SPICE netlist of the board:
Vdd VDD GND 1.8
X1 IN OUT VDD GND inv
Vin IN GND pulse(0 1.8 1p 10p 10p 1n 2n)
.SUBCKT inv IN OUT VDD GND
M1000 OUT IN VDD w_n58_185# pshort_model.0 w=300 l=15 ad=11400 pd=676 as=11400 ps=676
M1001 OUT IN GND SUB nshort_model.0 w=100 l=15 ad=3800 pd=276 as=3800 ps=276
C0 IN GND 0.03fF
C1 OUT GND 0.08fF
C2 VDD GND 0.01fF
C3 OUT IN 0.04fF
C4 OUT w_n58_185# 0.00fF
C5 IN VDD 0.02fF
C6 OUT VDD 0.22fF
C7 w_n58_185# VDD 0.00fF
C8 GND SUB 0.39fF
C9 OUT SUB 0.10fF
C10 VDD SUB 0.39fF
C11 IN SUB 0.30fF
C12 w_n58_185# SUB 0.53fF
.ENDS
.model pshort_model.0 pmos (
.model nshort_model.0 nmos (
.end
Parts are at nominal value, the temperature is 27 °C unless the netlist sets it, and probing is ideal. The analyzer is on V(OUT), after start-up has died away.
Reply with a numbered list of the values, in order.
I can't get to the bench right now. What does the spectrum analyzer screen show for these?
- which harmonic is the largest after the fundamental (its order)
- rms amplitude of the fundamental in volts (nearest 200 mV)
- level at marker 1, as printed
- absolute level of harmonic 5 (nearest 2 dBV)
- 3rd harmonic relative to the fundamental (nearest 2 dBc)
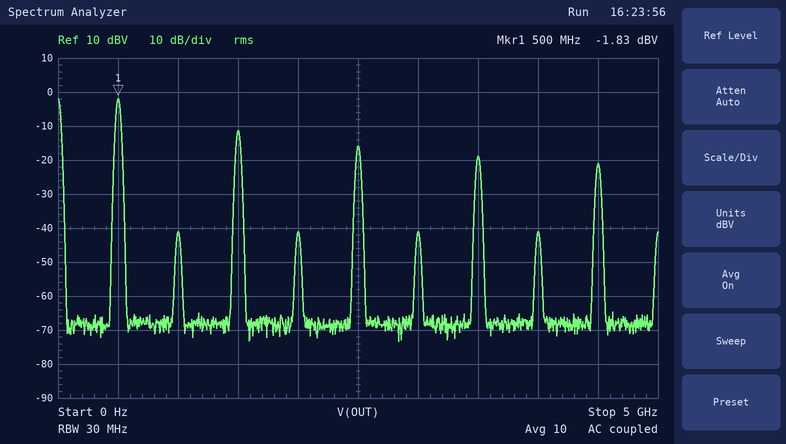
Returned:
1. 3
2. 800 mV
3. -1.83 dBV
4. -16 dBV
5. -10 dBc
